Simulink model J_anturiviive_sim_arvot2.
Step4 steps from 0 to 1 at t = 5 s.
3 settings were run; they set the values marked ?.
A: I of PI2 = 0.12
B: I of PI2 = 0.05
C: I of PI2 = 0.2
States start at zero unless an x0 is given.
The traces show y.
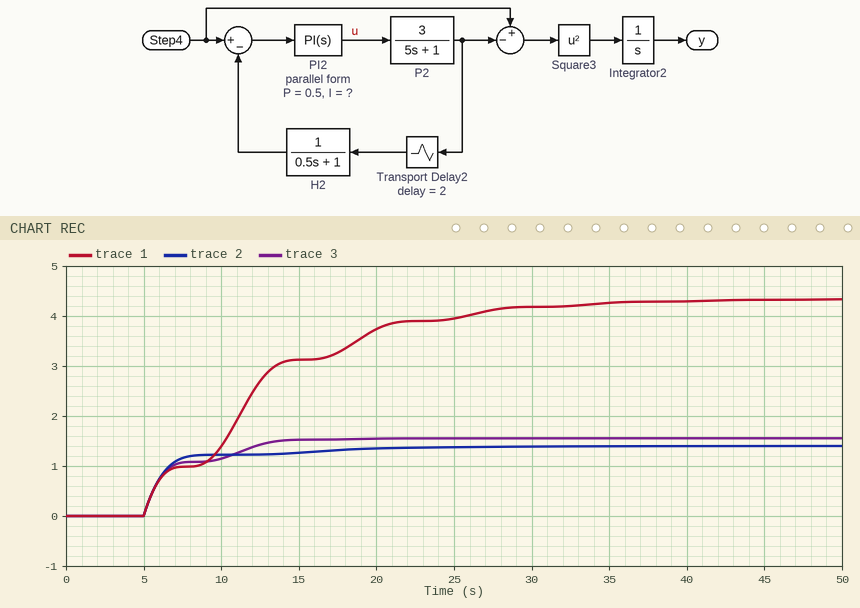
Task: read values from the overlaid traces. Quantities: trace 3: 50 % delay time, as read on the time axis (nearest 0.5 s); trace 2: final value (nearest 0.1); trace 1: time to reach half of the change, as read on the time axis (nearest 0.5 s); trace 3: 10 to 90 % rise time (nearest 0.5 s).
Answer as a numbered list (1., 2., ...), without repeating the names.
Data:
1. 6.0 s
2. 1.4
3. 11.5 s
4. 7.0 s
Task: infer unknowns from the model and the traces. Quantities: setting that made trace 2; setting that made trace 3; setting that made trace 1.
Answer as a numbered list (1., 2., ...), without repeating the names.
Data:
1. B
2. A
3. C
